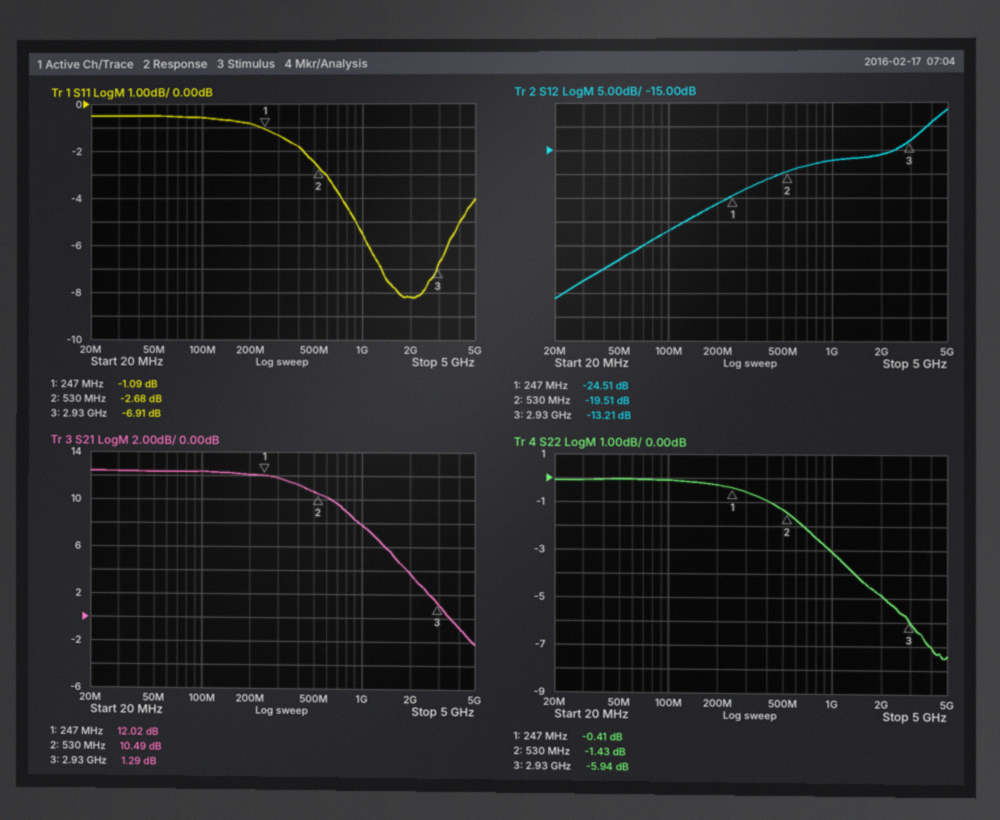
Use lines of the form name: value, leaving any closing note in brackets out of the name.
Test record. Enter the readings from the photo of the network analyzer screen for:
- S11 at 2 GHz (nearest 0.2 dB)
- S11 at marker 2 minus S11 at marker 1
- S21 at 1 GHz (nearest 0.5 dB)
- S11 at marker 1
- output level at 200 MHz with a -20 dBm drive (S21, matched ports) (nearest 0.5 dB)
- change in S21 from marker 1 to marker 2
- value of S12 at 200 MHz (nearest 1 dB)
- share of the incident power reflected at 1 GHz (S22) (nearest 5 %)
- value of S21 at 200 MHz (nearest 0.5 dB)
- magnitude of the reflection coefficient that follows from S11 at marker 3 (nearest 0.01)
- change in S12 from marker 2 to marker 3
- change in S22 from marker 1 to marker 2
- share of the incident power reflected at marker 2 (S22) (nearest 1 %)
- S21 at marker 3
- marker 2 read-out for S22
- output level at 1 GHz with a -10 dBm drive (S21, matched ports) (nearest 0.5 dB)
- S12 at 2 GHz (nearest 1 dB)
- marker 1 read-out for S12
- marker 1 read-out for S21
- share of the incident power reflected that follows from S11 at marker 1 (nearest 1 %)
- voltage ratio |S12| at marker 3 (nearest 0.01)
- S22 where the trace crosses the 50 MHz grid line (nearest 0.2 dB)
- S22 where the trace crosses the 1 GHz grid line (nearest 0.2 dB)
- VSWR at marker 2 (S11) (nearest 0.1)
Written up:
S11 at 2 GHz: -8.2 dB
S11 at marker 2 minus S11 at marker 1: -1.59 dB
S21 at 1 GHz: 8.0 dB
S11 at marker 1: -1.09 dB
output level at 200 MHz with a -20 dBm drive (S21, matched ports): -8.0 dBm
change in S21 from marker 1 to marker 2: -1.53 dB
value of S12 at 200 MHz: -26 dB
share of the incident power reflected at 1 GHz (S22): 50 %
value of S21 at 200 MHz: 12.0 dB
magnitude of the reflection coefficient that follows from S11 at marker 3: 0.45
change in S12 from marker 2 to marker 3: 6.30 dB
change in S22 from marker 1 to marker 2: -1.02 dB
share of the incident power reflected at marker 2 (S22): 72 %
S21 at marker 3: 1.29 dB
marker 2 read-out for S22: -1.43 dB
output level at 1 GHz with a -10 dBm drive (S21, matched ports): -2.0 dBm
S12 at 2 GHz: -16 dB
marker 1 read-out for S12: -24.51 dB
marker 1 read-out for S21: 12.02 dB
share of the incident power reflected that follows from S11 at marker 1: 78 %
voltage ratio |S12| at marker 3: 0.22
S22 where the trace crosses the 50 MHz grid line: 0.0 dB
S22 where the trace crosses the 1 GHz grid line: -3.0 dB
VSWR at marker 2 (S11): 6.5
